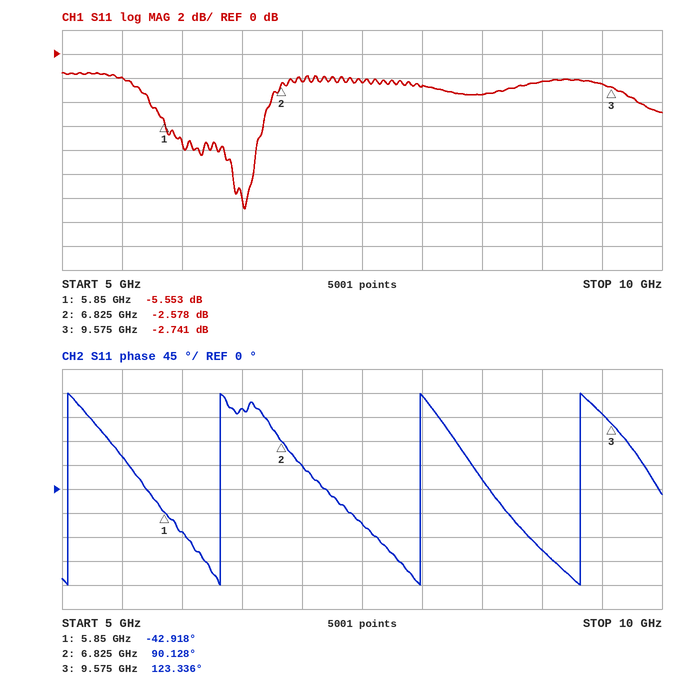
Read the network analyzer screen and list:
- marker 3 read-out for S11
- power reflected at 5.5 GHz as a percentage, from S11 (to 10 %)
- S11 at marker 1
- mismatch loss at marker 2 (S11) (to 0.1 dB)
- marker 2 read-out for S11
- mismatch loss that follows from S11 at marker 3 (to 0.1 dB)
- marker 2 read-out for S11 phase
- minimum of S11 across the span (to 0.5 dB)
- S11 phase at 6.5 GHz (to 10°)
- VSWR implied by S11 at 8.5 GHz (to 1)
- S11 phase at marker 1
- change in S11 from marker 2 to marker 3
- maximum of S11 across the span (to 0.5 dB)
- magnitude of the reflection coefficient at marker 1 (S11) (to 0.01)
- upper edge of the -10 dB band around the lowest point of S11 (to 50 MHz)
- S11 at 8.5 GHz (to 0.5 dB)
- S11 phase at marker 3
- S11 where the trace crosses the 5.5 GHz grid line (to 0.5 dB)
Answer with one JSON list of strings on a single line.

["-2.741 dB", "60 %", "-5.553 dB", "3.5 dB", "-2.578 dB", "3.3 dB", "90.128°", "-13.0 dB", "150°", "5", "-42.918°", "-0.163 dB", "-1.5 dB", "0.53", "6.60 GHz", "-3.5 dB", "123.336°", "-2.0 dB"]
